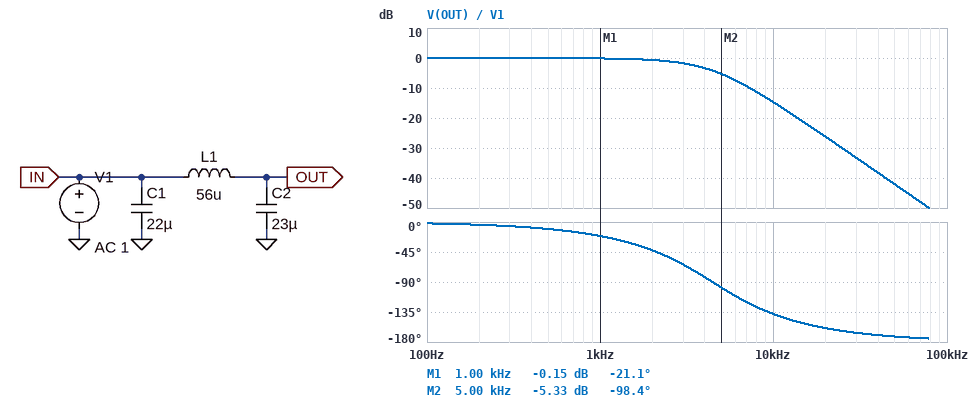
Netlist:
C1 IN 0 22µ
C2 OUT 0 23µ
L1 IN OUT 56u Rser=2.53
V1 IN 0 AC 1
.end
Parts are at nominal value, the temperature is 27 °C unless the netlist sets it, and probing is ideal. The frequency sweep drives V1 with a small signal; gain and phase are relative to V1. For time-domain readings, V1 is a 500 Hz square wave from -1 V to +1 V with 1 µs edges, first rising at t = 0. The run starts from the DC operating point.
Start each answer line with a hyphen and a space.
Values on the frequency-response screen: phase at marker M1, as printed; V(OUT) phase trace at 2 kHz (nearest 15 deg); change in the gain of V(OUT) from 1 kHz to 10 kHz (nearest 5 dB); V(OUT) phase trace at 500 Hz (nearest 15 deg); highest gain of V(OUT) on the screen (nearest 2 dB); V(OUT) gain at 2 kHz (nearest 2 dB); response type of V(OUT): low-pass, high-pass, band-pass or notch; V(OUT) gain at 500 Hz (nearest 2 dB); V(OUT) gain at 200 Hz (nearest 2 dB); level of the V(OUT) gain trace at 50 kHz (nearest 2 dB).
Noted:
- -21.1 deg
- -45 deg
- -15 dB
- -15 deg
- 0 dB
- 0 dB
- low-pass
- 0 dB
- 0 dB
- -42 dB
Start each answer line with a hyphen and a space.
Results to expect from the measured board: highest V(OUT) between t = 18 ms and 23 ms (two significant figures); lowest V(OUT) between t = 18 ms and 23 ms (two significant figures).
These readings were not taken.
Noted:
- 1.0 V
- -1.0 V
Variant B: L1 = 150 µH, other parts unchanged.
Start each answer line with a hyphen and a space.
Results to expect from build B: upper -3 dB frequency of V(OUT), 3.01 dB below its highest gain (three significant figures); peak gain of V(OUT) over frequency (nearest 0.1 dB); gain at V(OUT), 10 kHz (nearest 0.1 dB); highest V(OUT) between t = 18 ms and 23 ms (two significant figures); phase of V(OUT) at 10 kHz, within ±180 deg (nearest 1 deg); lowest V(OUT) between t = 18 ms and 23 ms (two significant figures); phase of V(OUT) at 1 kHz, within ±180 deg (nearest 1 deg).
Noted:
- 3.17 kHz
- 1.3 dB
- -22.4 dB
- 1.3 V
- -164 deg
- -1.3 V
- -23 deg
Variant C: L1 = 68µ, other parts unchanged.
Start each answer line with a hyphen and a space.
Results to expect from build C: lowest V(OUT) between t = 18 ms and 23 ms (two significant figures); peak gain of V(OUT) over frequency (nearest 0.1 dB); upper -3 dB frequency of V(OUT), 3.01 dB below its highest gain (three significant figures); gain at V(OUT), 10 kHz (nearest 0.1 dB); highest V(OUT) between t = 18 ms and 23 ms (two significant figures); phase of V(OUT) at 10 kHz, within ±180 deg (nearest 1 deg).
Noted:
- -1.1 V
- 0 dB
- 3.86 kHz
- -16.0 dB
- 1.1 V
- -145 deg
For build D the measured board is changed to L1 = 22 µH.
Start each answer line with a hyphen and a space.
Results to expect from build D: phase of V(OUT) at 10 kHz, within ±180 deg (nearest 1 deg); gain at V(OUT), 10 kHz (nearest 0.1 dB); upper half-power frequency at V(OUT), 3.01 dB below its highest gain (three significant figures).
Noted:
- -105 deg
- -11.6 dB
- 3.20 kHz
